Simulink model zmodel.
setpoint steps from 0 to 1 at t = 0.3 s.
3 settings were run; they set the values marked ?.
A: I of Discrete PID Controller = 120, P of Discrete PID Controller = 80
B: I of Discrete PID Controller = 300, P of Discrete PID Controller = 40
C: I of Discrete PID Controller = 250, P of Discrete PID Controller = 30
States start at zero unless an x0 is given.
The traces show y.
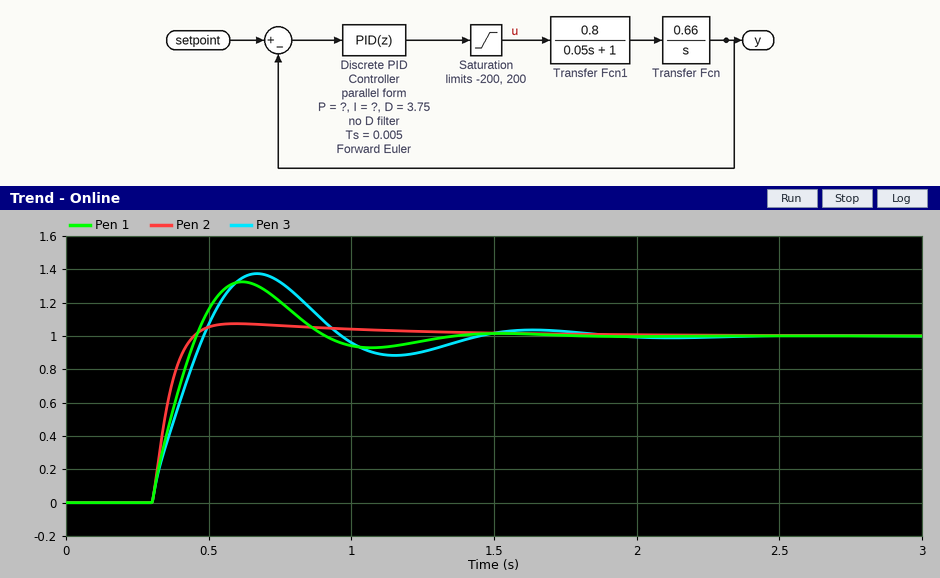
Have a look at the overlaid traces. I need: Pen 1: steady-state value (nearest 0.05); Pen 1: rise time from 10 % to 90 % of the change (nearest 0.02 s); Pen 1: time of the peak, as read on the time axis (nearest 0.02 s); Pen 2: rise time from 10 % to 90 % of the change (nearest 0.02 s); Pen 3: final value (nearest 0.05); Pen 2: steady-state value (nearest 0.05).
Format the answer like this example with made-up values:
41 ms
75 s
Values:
1.00
0.12 s
0.62 s
0.10 s
1.00
1.00
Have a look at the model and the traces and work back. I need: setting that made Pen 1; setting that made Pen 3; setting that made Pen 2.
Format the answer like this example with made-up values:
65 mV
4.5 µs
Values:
B
C
A
